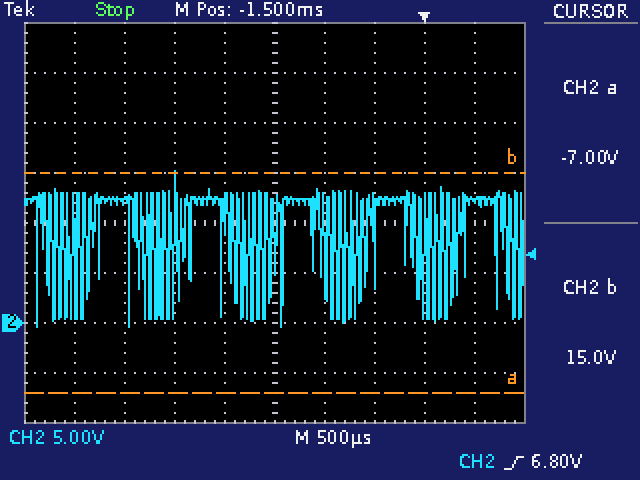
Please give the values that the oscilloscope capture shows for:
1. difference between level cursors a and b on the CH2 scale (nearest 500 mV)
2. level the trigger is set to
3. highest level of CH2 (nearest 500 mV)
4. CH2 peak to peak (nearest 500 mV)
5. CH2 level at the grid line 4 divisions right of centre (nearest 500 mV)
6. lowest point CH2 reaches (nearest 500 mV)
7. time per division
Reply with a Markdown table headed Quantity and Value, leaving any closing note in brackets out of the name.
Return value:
| Quantity | Value |
|---|---|
| difference between level cursors a and b on the CH2 scale | 22.0 V |
| level the trigger is set to | 6.80 V |
| highest level of CH2 | 15.0 V |
| CH2 peak to peak | 15.5 V |
| CH2 level at the grid line 4 divisions right of centre | 12.5 V |
| lowest point CH2 reaches | -500 mV |
| time per division | 500 µs |
